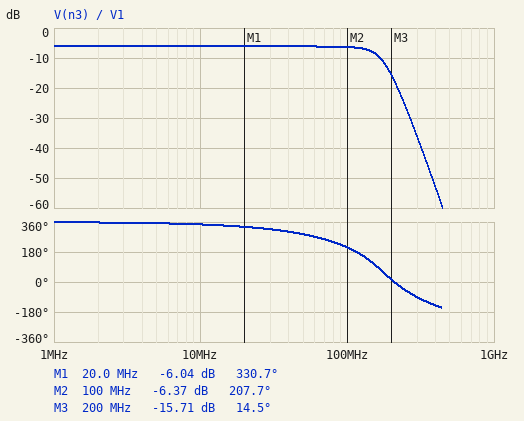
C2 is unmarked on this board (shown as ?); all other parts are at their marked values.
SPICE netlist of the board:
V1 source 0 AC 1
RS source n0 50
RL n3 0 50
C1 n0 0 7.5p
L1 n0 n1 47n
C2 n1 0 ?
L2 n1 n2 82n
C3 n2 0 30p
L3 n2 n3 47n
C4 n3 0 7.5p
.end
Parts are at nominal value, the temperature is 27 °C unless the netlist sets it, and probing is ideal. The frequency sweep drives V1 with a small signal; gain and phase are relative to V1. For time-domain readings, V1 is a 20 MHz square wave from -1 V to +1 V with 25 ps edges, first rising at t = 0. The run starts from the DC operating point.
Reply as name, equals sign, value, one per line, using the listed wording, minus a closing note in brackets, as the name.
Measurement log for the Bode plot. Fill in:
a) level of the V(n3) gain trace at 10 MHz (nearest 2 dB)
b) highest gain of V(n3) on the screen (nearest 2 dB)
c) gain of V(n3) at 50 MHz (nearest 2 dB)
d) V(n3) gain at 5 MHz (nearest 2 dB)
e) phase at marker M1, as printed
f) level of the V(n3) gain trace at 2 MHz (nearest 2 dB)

level of the V(n3) gain trace at 10 MHz = -6 dB
highest gain of V(n3) on the screen = -6 dB
gain of V(n3) at 50 MHz = -6 dB
V(n3) gain at 5 MHz = -6 dB
phase at marker M1, as printed = 330.7 deg
level of the V(n3) gain trace at 2 MHz = -6 dB
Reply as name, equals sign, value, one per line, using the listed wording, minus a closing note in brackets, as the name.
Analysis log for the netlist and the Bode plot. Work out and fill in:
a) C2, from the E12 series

C2, from the E12 series = 47 pF
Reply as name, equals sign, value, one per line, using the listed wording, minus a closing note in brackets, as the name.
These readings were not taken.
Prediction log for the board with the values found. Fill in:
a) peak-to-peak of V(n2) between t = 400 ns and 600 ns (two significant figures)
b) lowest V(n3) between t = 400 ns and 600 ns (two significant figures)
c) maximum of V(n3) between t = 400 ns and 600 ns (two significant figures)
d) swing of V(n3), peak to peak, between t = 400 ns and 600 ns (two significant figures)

peak-to-peak of V(n2) between t = 400 ns and 600 ns = 1.3 V
lowest V(n3) between t = 400 ns and 600 ns = -620 mV
maximum of V(n3) between t = 400 ns and 600 ns = 620 mV
swing of V(n3), peak to peak, between t = 400 ns and 600 ns = 1.2 V
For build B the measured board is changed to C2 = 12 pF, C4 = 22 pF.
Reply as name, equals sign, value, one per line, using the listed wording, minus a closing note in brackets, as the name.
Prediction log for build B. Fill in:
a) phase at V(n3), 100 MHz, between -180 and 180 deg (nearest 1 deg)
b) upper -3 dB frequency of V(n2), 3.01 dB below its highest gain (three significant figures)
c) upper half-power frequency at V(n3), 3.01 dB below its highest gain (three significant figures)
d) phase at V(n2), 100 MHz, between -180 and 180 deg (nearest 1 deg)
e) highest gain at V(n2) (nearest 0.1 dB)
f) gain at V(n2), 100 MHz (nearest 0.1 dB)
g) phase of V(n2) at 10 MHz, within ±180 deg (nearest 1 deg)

phase at V(n3), 100 MHz, between -180 and 180 deg = -130 deg
upper -3 dB frequency of V(n2), 3.01 dB below its highest gain = 267 MHz
upper half-power frequency at V(n3), 3.01 dB below its highest gain = 218 MHz
phase at V(n2), 100 MHz, between -180 and 180 deg = -85 deg
highest gain at V(n2) = -4.8 dB
gain at V(n2), 100 MHz = -8.8 dB
phase of V(n2) at 10 MHz, within ±180 deg = -9 deg
